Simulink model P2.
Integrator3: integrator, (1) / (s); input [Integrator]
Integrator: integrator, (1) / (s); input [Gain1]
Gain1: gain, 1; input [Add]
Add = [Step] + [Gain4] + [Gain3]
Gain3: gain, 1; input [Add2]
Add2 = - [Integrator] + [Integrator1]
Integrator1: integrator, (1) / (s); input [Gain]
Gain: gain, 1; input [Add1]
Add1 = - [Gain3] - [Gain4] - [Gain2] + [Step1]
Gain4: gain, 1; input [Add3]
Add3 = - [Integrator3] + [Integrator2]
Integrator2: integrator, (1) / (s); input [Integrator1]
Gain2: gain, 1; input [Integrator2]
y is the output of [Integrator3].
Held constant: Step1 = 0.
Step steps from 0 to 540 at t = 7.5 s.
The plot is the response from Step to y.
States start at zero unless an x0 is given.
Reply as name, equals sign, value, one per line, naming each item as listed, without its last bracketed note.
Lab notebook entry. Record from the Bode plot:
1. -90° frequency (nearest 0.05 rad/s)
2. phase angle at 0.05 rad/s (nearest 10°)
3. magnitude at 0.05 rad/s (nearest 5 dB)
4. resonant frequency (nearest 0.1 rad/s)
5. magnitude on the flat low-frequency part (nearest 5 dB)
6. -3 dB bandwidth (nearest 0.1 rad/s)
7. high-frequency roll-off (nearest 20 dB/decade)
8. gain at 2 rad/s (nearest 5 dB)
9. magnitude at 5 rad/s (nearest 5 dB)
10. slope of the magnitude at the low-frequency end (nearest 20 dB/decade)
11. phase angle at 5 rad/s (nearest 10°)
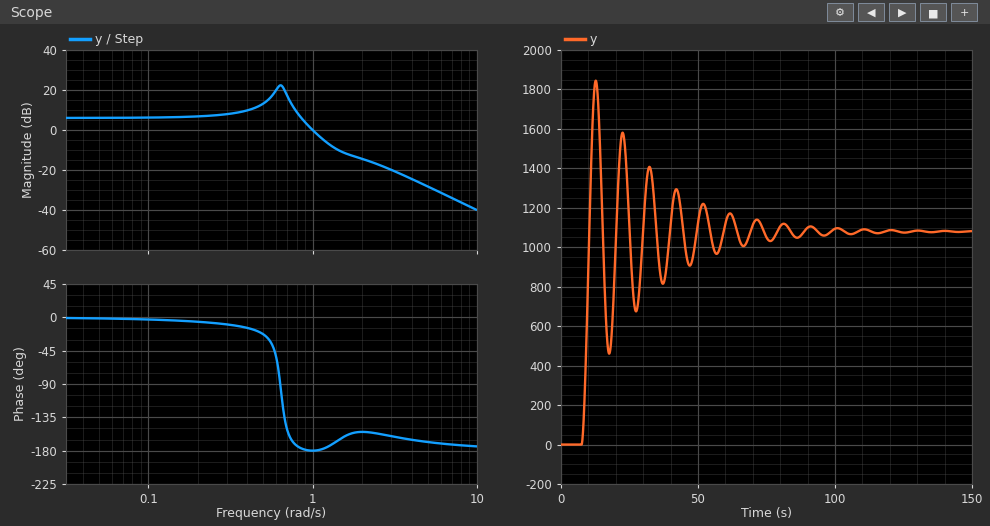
-90° frequency = 0.65 rad/s
phase angle at 0.05 rad/s = 0°
magnitude at 0.05 rad/s = 5 dB
resonant frequency = 0.6 rad/s
magnitude on the flat low-frequency part = 5 dB
-3 dB bandwidth = 0.9 rad/s
high-frequency roll-off = -40 dB/decade
gain at 2 rad/s = -15 dB
magnitude at 5 rad/s = -30 dB
slope of the magnitude at the low-frequency end = 0 dB/decade
phase angle at 5 rad/s = -170°
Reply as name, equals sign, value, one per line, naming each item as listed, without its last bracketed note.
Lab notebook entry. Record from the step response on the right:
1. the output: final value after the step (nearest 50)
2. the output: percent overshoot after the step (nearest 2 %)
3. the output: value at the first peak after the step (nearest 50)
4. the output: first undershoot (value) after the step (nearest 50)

the output: final value after the step = 1100
the output: percent overshoot after the step = 70 %
the output: value at the first peak after the step = 1850
the output: first undershoot (value) after the step = 450
